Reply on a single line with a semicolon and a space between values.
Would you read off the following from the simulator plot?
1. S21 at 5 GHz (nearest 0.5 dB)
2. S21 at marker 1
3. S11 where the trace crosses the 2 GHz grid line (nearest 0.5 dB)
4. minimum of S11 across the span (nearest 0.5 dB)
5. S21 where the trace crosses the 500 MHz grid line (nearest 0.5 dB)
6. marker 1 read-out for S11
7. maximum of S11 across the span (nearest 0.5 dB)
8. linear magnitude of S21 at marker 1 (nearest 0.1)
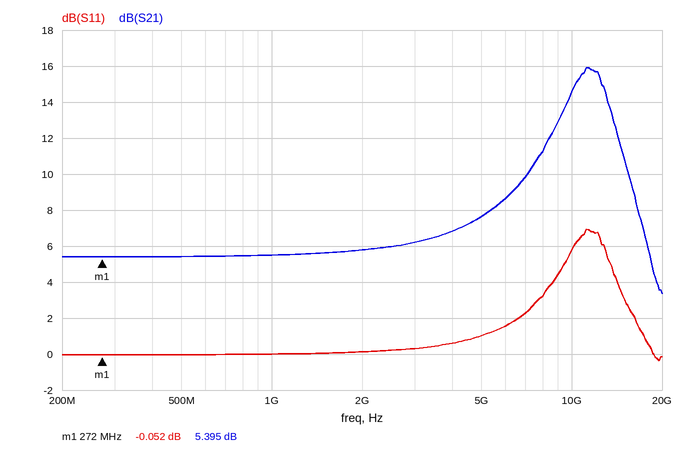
7.5 dB; 5.395 dB; 0.0 dB; -0.5 dB; 5.5 dB; -0.052 dB; 7.0 dB; 1.9
